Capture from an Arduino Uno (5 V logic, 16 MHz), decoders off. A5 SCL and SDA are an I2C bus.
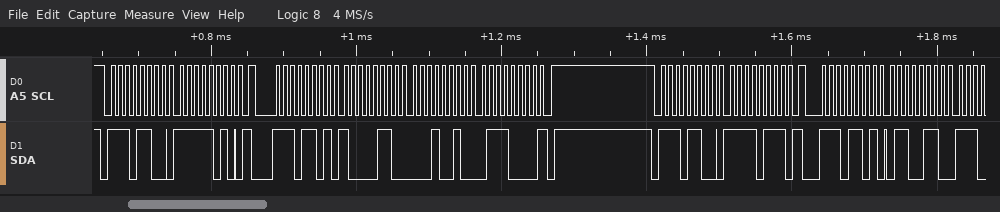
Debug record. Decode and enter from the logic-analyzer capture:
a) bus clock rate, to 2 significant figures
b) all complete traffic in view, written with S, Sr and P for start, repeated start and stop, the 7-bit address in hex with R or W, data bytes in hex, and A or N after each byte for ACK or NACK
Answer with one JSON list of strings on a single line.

["100 kHz", "S 76W A FA A Sr 76R A 86 A 12 A 70 N P S 76W A F7 A Sr 76R A 66 A"]
